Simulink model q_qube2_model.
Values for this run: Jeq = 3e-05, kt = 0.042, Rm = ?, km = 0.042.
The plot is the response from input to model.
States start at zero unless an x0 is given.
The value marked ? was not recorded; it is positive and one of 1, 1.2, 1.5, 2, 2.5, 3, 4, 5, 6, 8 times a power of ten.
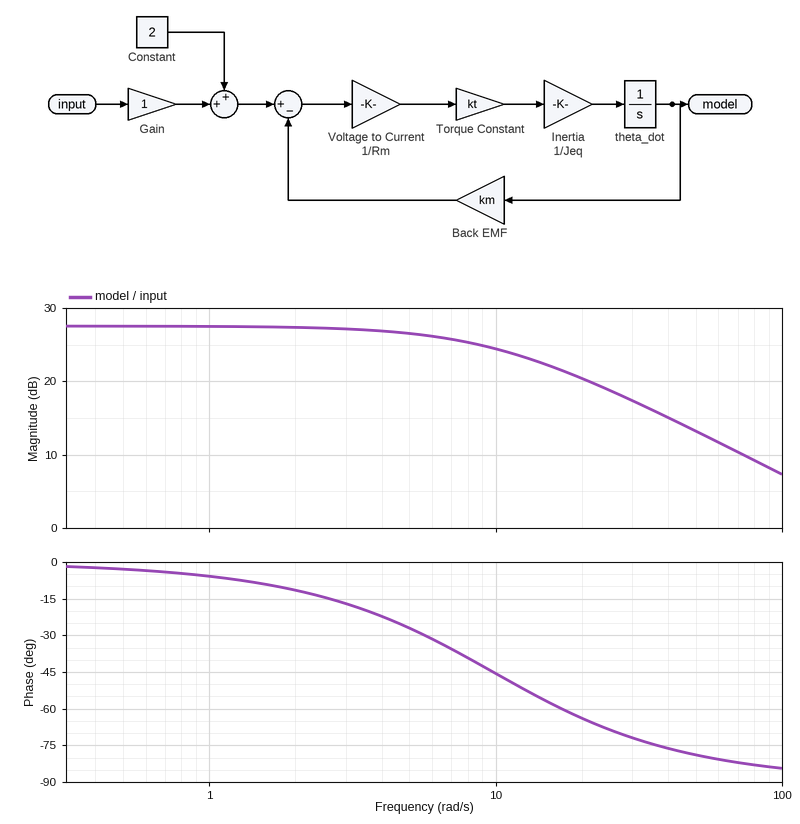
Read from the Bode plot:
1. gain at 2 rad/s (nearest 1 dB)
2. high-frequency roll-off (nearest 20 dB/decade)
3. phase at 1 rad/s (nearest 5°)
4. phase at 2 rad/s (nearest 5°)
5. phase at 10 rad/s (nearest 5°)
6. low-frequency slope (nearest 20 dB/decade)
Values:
27 dB
-20 dB/decade
-5°
-10°
-45°
0 dB/decade
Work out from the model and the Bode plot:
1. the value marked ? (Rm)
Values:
6
